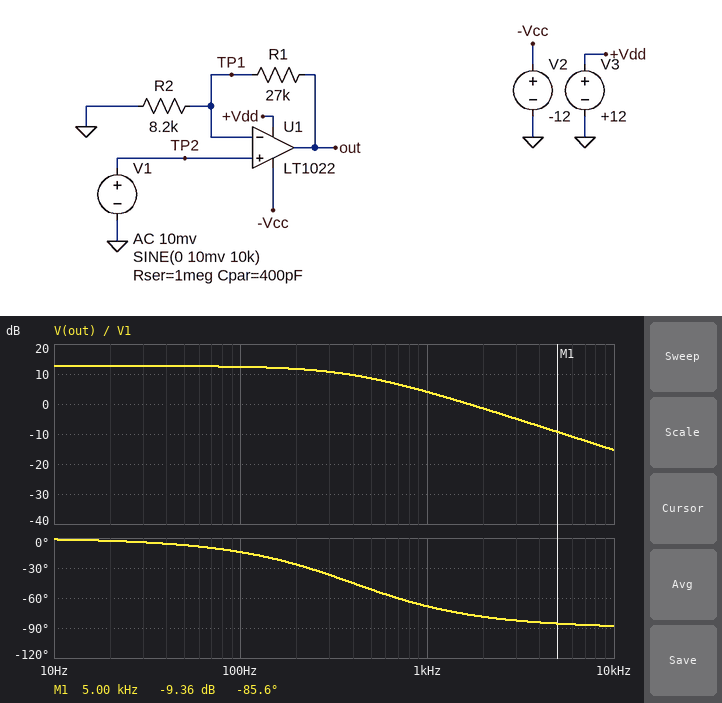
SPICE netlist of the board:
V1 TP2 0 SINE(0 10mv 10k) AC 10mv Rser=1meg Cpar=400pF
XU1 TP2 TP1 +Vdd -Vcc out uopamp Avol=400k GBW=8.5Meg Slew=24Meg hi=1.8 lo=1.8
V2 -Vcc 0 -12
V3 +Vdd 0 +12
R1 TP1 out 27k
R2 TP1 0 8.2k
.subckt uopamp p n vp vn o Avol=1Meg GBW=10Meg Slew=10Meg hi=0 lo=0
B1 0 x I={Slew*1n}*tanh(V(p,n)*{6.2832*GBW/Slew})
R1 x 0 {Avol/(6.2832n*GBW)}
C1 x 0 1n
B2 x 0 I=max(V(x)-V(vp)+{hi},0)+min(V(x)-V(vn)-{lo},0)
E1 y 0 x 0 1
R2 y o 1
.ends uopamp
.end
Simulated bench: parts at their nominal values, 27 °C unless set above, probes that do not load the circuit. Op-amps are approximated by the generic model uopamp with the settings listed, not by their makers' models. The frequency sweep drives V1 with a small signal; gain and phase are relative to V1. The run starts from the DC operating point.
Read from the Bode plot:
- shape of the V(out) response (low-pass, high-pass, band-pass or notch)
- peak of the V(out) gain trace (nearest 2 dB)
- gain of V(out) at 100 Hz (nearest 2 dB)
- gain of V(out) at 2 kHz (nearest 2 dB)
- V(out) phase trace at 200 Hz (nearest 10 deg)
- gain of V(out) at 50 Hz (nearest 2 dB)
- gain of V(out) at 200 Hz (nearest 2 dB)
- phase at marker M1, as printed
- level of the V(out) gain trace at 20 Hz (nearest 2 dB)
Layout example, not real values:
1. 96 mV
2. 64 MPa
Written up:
1. low-pass
2. 12 dB
3. 12 dB
4. -2 dB
5. -30 deg
6. 12 dB
7. 12 dB
8. -85.6 deg
9. 12 dB
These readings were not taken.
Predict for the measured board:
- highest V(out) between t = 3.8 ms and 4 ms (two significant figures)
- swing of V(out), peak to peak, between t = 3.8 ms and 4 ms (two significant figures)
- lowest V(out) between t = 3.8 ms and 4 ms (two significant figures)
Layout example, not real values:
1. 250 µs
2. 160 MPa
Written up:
1. 1.7 mV
2. 3.4 mV
3. -1.7 mV
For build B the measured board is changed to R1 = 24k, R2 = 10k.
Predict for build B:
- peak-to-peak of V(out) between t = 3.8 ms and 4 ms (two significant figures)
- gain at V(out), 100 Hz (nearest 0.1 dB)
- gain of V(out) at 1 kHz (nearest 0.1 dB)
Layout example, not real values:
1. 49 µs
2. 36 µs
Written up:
1. 2.7 mV
2. 10.4 dB
3. 2.0 dB
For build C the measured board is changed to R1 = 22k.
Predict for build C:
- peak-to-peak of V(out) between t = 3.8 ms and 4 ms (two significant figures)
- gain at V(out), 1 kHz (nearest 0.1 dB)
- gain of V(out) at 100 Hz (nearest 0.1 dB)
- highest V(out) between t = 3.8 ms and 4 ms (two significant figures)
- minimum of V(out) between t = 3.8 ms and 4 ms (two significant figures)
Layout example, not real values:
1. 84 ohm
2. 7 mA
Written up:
1. 2.9 mV
2. 2.7 dB
3. 11.1 dB
4. 1.5 mV
5. -1.5 mV
